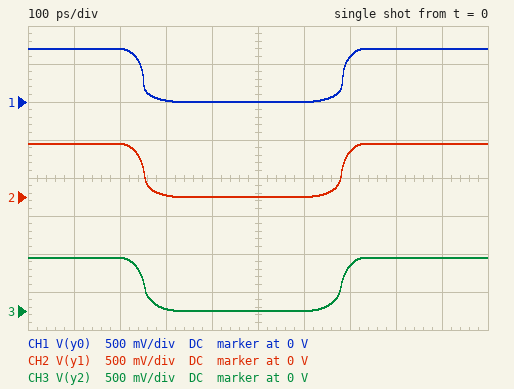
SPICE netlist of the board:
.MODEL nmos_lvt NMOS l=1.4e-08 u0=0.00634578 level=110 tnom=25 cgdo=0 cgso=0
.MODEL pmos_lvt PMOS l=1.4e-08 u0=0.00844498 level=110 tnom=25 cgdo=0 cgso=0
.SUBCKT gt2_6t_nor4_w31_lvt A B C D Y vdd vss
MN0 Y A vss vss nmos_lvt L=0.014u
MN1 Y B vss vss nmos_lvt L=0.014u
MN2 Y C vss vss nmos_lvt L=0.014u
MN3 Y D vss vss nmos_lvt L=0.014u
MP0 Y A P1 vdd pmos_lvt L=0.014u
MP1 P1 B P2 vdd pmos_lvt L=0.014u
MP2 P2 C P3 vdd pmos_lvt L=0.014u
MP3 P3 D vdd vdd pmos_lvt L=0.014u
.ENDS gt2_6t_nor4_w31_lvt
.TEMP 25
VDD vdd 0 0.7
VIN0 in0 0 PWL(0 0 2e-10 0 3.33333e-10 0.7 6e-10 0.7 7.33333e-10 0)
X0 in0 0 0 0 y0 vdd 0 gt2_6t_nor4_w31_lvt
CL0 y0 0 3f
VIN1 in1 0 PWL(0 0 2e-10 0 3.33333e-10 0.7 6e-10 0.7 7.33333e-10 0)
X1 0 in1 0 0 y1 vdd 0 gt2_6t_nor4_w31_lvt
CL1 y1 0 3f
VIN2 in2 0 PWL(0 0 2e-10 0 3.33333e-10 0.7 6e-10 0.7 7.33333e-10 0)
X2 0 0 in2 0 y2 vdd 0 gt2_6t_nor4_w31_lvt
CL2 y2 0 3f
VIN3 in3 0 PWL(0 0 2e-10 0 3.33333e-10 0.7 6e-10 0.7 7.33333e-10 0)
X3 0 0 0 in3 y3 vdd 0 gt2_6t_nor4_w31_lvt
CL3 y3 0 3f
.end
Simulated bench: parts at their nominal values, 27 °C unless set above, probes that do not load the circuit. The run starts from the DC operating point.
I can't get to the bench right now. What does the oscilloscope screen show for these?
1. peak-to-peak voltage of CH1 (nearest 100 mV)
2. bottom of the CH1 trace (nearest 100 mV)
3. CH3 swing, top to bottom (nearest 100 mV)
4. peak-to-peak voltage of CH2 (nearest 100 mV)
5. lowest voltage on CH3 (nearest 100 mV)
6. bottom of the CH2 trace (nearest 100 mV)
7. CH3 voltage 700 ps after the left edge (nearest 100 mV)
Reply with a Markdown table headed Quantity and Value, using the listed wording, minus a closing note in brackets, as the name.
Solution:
| Quantity | Value |
|---|---|
| peak-to-peak voltage of CH1 | 700 mV |
| bottom of the CH1 trace | 0 V |
| CH3 swing, top to bottom | 700 mV |
| peak-to-peak voltage of CH2 | 700 mV |
| lowest voltage on CH3 | 0 V |
| bottom of the CH2 trace | 0 V |
| CH3 voltage 700 ps after the left edge | 600 mV |
